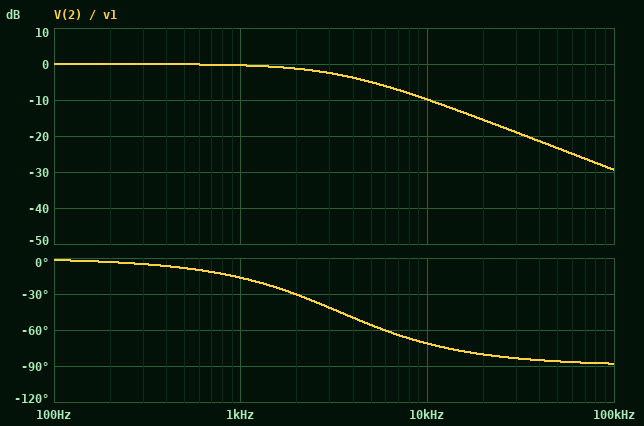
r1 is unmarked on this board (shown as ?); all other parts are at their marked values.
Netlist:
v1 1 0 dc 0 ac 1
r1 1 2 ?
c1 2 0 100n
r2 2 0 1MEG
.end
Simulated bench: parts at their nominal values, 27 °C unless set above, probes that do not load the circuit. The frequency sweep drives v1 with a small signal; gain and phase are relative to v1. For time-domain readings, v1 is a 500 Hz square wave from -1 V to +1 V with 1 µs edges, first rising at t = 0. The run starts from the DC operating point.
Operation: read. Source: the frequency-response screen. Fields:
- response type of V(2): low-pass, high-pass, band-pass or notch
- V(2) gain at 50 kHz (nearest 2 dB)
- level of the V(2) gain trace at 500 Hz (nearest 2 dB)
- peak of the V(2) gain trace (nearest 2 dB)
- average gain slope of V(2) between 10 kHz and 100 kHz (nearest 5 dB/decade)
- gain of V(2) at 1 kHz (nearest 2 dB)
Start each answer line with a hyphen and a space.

- low-pass
- -24 dB
- 0 dB
- 0 dB
- -20 dB/decade
- 0 dB
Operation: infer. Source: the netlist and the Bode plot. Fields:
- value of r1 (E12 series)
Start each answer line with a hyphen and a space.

- 470 Ω
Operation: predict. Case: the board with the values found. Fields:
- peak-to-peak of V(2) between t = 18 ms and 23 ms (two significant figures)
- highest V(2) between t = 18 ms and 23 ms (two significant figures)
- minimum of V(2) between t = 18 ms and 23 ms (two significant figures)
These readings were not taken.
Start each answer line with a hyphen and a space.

- 2.0 V
- 1.0 V
- -1.0 V
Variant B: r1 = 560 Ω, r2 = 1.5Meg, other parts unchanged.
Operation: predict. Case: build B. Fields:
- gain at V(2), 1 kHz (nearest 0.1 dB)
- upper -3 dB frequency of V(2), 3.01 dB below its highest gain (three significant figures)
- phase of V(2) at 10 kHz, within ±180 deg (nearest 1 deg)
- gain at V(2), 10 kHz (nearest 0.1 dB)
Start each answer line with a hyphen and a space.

- -0.5 dB
- 2.84 kHz
- -74 deg
- -11.3 dB
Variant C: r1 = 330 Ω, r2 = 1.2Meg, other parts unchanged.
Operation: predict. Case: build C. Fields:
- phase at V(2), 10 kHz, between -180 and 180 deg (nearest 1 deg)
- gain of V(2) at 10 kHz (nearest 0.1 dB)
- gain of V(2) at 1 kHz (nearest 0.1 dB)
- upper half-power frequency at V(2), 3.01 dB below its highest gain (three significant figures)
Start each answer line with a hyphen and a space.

- -64 deg
- -7.2 dB
- -0.2 dB
- 4.82 kHz
